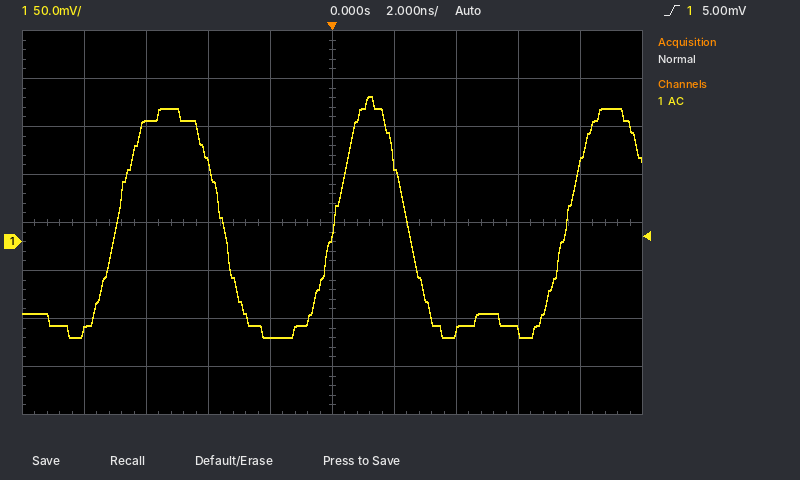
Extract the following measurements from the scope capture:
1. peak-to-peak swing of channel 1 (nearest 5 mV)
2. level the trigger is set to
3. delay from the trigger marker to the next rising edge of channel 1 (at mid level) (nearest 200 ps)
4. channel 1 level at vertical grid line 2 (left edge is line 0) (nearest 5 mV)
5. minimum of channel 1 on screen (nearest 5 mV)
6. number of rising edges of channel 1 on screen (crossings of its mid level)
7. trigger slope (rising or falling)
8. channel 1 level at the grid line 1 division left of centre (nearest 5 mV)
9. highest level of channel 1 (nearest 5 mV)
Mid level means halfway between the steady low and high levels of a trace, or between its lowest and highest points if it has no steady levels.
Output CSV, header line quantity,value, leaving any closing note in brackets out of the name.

quantity,value
peak-to-peak swing of channel 1,250 mV
level the trigger is set to,5.00 mV
delay from the trigger marker to the next rising edge of channel 1 (at mid level),7.6 ns
channel 1 level at vertical grid line 2 (left edge is line 0),125 mV
minimum of channel 1 on screen,-100 mV
number of rising edges of channel 1 on screen,3
trigger slope,rising
channel 1 level at the grid line 1 division left of centre,-100 mV
highest level of channel 1,150 mV
